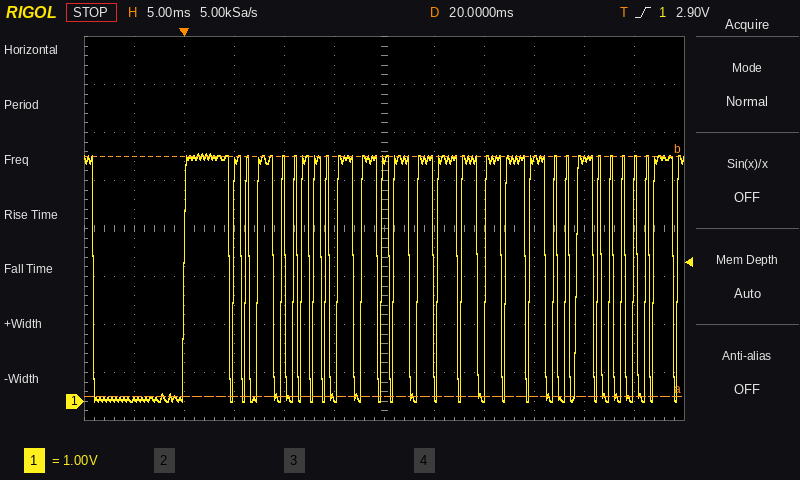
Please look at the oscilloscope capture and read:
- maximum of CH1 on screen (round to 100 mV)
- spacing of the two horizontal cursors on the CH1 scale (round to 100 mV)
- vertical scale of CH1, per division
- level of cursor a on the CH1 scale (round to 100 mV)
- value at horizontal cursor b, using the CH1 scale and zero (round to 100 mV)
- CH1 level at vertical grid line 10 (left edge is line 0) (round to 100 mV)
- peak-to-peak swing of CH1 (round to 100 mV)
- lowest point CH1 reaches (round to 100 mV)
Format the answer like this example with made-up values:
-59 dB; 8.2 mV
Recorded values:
5.2 V; 5.0 V; 1 V; 100 mV; 5.1 V; 5.0 V; 5.2 V; 0.0 V
